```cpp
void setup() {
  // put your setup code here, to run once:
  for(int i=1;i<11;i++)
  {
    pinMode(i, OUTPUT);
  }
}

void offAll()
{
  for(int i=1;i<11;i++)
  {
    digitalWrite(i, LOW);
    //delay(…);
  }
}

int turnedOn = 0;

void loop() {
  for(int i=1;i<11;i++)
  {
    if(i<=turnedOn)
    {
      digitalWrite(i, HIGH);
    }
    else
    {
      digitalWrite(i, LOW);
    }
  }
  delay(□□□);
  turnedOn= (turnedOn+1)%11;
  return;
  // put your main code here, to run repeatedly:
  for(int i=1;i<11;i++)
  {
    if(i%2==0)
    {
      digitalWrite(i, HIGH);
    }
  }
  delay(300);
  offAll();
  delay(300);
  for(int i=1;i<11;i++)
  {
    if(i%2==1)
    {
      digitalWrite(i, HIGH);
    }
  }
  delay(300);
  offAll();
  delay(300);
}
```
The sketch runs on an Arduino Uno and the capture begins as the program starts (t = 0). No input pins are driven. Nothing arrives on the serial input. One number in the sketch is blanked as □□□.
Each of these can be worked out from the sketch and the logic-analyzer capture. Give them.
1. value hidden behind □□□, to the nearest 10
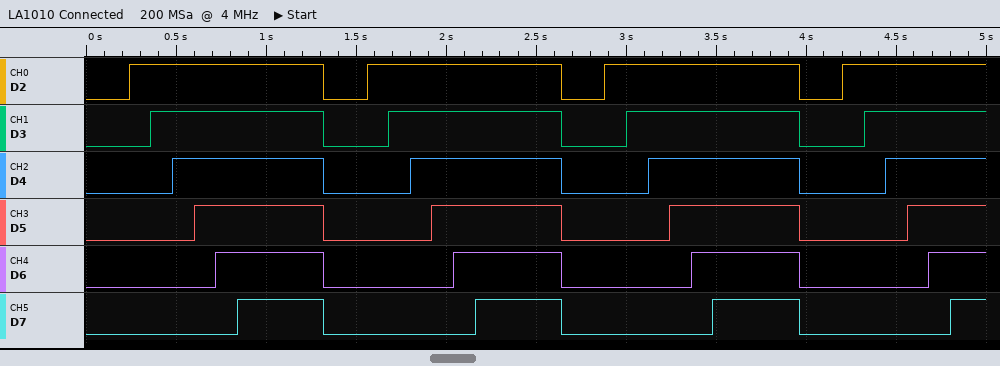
120
